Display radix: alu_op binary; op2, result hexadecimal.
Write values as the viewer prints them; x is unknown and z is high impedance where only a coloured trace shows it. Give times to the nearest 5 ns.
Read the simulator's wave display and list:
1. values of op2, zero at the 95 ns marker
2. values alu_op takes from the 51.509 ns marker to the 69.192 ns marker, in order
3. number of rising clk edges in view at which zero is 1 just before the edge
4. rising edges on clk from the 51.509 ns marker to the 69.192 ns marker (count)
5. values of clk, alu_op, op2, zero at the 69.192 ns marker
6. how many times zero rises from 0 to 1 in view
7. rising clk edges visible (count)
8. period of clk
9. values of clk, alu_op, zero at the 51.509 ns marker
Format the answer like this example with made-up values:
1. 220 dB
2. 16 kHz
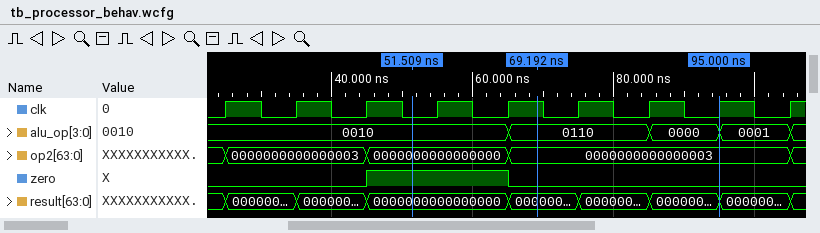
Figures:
1. op2=0000000000000003, zero=0
2. 0010, 0110
3. 2
4. 2
5. clk=1, alu_op=0110, op2=0000000000000003, zero=0
6. 1
7. 9
8. 10 ns
9. clk=0, alu_op=0010, zero=1
